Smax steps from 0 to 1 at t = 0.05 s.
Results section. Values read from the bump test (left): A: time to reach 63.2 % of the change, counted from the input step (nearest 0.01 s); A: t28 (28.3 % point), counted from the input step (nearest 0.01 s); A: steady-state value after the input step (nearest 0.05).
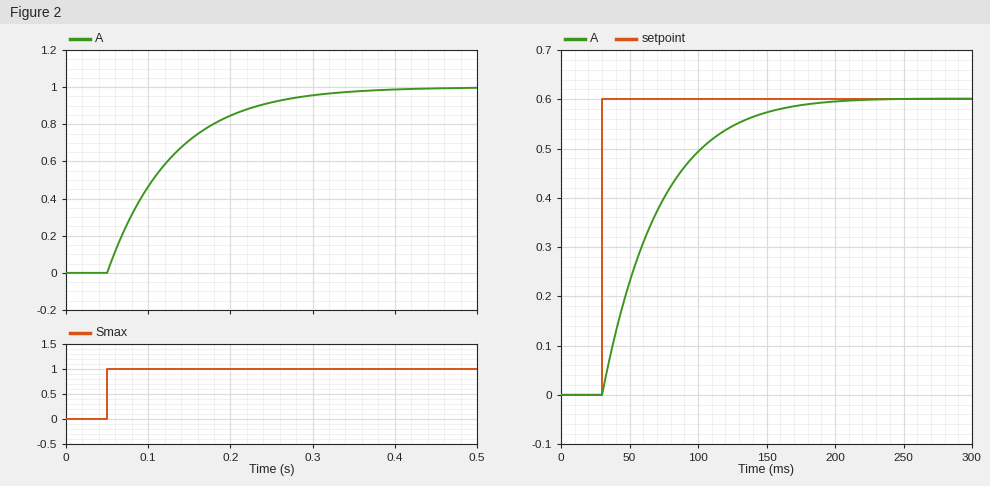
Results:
0.08 s
0.03 s
1.00
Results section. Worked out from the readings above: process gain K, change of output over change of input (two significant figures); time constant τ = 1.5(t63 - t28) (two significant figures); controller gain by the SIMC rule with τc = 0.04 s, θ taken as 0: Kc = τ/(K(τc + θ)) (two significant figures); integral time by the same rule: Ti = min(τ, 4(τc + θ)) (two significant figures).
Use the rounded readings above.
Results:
1.0
0.075 s
1.9
0.075 s
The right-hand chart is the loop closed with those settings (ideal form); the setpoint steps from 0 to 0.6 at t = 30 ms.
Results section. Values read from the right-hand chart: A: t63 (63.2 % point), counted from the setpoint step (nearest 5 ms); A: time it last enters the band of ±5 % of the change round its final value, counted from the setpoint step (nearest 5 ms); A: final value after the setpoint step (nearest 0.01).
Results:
40 ms
115 ms
0.60
